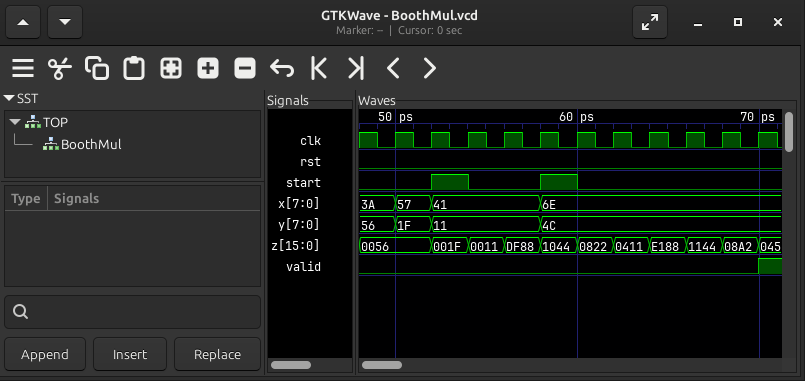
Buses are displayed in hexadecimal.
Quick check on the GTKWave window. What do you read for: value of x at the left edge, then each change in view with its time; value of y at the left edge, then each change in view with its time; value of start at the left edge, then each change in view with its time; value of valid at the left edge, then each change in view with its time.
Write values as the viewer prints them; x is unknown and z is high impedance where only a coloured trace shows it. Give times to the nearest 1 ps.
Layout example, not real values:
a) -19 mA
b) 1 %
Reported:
a) 3A, 57 at 50 ps, 41 at 52 ps, 6E at 58 ps
b) 56, 1F at 50 ps, 11 at 52 ps, 4C at 58 ps
c) 0, 1 at 52 ps, 0 at 54 ps, 1 at 58 ps, 0 at 60 ps
d) 0, 1 at 70 ps
